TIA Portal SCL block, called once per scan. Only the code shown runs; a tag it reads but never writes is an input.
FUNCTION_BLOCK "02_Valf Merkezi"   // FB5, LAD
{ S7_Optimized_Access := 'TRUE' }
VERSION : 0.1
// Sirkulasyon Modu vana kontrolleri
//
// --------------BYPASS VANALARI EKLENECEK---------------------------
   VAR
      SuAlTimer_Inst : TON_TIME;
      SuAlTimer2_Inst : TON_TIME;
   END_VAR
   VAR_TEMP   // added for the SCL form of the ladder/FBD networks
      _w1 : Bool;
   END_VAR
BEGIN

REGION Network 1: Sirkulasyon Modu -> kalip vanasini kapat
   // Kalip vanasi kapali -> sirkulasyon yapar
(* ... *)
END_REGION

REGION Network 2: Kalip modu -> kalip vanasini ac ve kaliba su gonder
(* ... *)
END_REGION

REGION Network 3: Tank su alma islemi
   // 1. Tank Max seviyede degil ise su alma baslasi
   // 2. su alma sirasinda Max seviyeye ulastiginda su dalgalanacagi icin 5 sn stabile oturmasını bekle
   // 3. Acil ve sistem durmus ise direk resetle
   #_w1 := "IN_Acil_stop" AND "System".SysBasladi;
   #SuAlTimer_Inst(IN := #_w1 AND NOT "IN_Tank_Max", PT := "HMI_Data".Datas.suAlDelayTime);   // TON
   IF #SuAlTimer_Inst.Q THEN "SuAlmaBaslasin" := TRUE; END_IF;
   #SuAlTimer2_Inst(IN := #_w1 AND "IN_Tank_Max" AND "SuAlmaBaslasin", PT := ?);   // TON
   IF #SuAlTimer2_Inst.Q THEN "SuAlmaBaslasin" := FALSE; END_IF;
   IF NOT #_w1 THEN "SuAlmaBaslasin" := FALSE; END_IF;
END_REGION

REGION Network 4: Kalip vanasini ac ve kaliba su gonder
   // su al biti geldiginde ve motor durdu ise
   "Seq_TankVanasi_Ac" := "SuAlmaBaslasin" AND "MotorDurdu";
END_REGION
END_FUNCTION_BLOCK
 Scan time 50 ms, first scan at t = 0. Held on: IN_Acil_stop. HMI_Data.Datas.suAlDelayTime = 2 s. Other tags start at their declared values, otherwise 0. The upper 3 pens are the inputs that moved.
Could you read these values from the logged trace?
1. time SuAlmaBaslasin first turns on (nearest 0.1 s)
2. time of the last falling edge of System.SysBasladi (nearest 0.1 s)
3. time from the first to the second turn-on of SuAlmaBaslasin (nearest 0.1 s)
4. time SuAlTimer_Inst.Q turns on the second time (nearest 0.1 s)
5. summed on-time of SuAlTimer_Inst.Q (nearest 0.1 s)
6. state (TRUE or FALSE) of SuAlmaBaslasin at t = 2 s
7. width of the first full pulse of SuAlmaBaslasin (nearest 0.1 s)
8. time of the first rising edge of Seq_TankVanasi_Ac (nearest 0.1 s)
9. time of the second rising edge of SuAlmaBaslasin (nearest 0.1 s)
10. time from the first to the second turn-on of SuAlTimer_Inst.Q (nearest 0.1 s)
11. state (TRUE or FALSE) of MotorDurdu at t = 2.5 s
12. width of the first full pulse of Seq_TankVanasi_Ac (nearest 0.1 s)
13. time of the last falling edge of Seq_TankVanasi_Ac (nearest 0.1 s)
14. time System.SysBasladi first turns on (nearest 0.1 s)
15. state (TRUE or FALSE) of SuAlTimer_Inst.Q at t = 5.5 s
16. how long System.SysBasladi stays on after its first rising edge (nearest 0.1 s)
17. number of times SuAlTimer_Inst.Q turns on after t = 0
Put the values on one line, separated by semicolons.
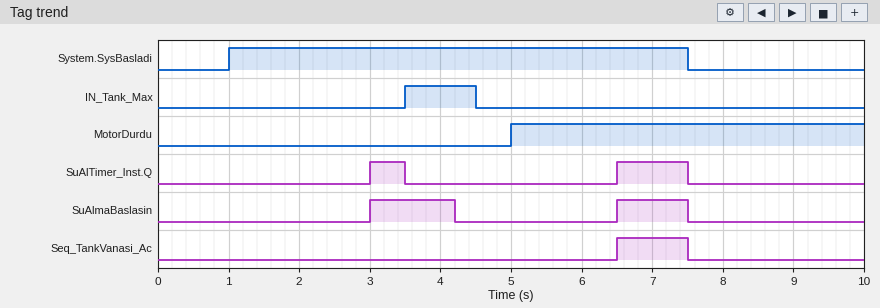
3.0 s; 7.5 s; 3.5 s; 6.5 s; 1.5 s; FALSE; 1.2 s; 6.5 s; 6.5 s; 3.5 s; FALSE; 1.0 s; 7.5 s; 1.0 s; FALSE; 6.5 s; 2
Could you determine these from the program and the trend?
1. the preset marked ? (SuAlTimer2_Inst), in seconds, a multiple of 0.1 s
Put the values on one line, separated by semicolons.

0.7 s
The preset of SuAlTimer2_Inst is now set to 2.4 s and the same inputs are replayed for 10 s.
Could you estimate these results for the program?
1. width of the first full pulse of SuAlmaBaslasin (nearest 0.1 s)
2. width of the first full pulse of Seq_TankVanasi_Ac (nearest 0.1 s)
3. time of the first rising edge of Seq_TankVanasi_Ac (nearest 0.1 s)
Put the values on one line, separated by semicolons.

4.5 s; 2.5 s; 5.0 s
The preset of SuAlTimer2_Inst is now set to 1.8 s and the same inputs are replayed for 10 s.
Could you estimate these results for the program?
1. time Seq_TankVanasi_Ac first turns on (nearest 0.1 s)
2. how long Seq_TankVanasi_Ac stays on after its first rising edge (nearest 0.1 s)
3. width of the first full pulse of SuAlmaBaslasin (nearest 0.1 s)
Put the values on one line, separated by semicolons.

5.0 s; 2.5 s; 4.5 s
